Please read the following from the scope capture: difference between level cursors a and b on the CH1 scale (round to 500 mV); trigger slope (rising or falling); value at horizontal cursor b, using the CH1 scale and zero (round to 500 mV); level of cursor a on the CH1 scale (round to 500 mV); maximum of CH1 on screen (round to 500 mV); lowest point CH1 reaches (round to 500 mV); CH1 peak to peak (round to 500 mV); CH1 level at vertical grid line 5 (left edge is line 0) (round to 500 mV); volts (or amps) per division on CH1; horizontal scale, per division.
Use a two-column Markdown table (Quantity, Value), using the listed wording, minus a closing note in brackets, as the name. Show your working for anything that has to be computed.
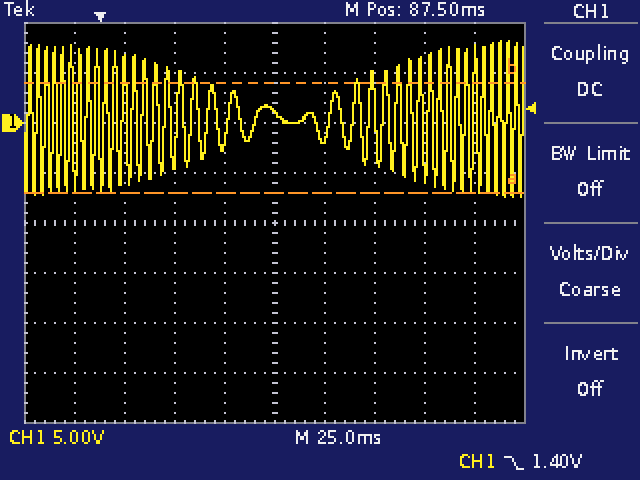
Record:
| Quantity | Value |
|---|---|
| difference between level cursors a and b on the CH1 scale | 11.0 V |
| trigger slope | falling |
| value at horizontal cursor b, using the CH1 scale and zero | 4.0 V |
| level of cursor a on the CH1 scale | -7.0 V |
| maximum of CH1 on screen | 8.0 V |
| lowest point CH1 reaches | -7.5 V |
| CH1 peak to peak | 8.0 V − (-7.5 V) = 15.5 V |
| CH1 level at vertical grid line 5 (left edge is line 0) | 1.0 V |
| volts (or amps) per division on CH1 | 5 V |
| horizontal scale, per division | 25 ms |
